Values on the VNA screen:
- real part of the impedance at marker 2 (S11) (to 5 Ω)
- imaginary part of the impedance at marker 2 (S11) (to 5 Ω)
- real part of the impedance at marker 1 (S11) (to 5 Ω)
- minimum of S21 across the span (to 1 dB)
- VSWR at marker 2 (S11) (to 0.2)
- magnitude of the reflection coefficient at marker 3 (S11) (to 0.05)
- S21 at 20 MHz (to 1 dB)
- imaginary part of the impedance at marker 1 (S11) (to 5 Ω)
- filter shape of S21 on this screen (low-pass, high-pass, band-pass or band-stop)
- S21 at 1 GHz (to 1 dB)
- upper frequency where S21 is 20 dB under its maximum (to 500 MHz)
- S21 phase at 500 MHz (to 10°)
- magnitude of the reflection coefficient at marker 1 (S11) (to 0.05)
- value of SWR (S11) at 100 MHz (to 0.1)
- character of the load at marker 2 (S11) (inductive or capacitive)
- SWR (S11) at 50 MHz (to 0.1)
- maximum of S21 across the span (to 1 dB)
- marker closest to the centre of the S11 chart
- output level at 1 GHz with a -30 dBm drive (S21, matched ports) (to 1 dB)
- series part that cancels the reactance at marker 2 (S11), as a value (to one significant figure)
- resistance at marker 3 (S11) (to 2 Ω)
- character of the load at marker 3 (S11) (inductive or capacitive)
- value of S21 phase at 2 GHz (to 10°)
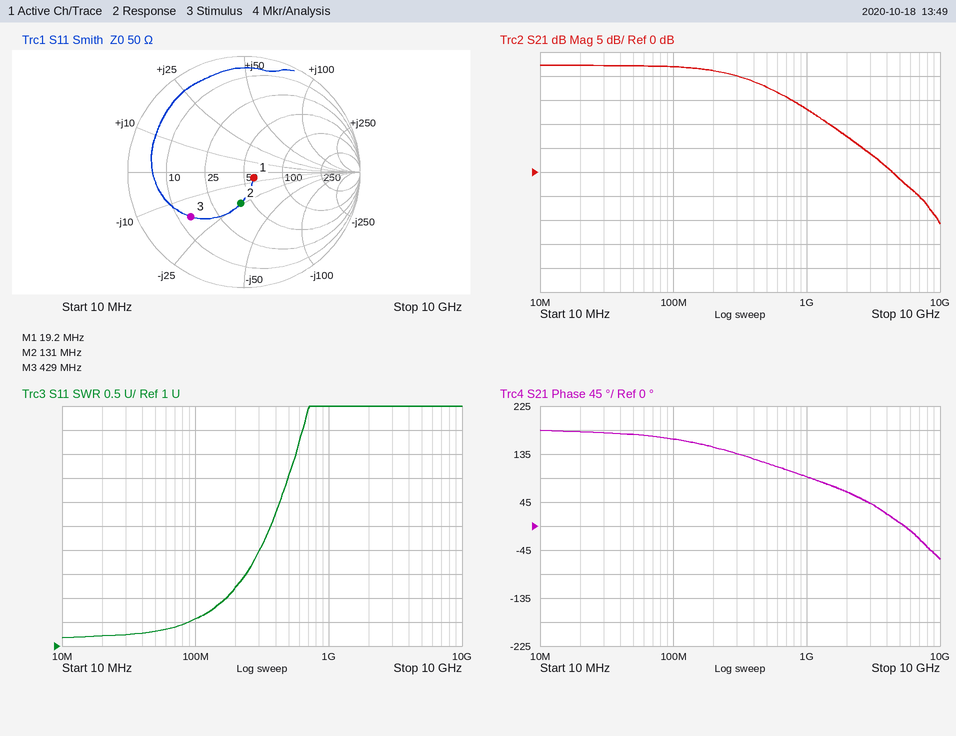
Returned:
40 Ω
-25 Ω
60 Ω
-11 dB
1.8
0.60
22 dB
-5 Ω
low-pass
13 dB
3.5 GHz
120°
0.10
1.6
capacitive
1.3
22 dB
marker 1
-17 dBm
30 nH
14 Ω
capacitive
60°
